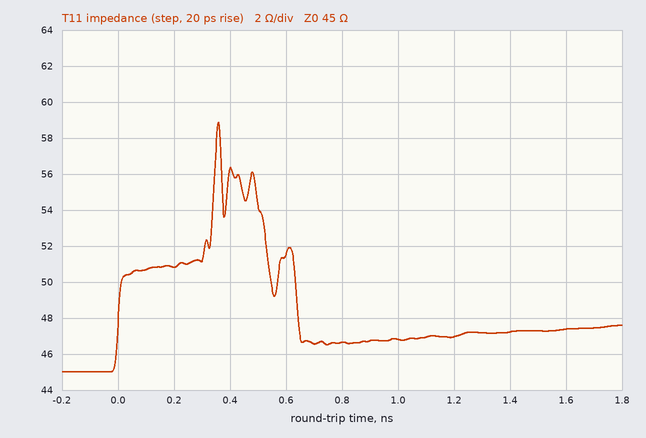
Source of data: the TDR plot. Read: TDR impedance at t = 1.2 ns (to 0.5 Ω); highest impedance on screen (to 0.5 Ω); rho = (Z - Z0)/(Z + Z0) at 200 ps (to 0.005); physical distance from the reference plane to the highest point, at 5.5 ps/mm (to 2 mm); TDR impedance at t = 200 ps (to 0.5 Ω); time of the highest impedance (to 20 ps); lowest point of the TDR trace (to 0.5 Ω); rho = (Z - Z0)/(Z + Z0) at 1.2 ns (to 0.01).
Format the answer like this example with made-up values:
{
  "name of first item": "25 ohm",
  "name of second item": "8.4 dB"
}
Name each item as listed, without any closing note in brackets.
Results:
{
  "TDR impedance at t = 1.2 ns": "47.0 Ω",
  "highest impedance on screen": "59.0 Ω",
  "rho = (Z - Z0)/(Z + Z0) at 200 ps": "+0.060",
  "physical distance from the reference plane to the highest point, at 5.5 ps/mm": "32 mm",
  "TDR impedance at t = 200 ps": "51.0 Ω",
  "time of the highest impedance": "360 ps",
  "lowest point of the TDR trace": "45.0 Ω",
  "rho = (Z - Z0)/(Z + Z0) at 1.2 ns": "+0.02"
}
